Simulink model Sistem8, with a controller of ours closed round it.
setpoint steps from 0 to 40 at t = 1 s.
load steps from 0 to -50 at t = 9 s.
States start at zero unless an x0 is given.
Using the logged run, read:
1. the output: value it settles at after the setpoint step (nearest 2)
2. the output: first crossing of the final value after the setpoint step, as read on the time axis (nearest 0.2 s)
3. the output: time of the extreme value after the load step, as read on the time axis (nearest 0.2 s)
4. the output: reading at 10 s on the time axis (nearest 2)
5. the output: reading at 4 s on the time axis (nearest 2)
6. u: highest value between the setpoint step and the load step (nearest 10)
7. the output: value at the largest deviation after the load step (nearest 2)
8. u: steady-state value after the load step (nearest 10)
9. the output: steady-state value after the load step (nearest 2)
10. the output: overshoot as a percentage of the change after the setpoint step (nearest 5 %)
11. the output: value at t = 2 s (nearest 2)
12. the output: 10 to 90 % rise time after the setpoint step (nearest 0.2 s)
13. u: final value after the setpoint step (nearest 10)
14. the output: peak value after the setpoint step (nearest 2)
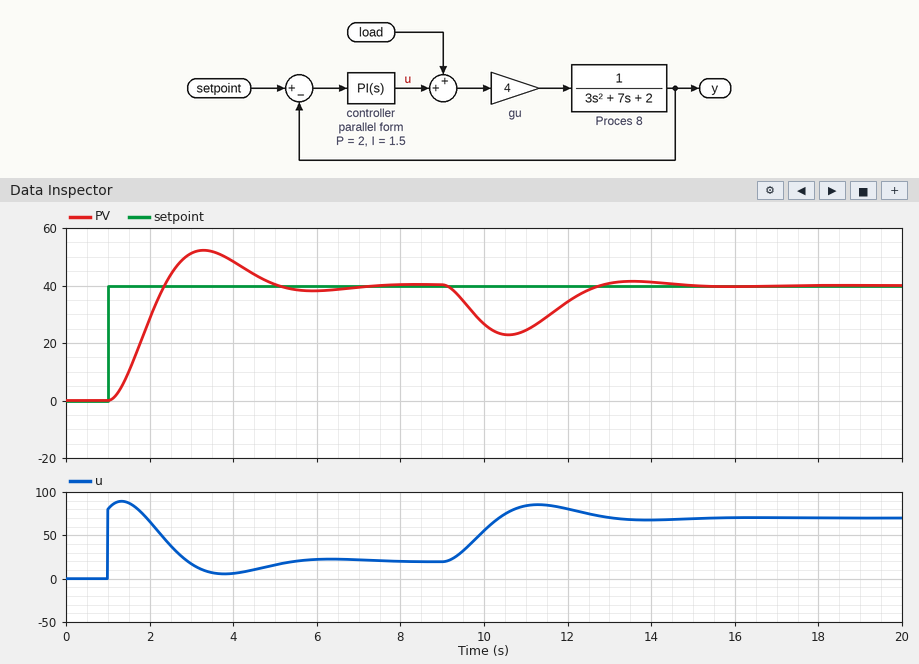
40
2.4 s
10.6 s
26
48
90
22
70
40
30 %
28
1.0 s
20
52
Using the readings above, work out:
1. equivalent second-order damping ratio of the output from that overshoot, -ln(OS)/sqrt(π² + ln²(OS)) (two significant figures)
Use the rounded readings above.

0.36
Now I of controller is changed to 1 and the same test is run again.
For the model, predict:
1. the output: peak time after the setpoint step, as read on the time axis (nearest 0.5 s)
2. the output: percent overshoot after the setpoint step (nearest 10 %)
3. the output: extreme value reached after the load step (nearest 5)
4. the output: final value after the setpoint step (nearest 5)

3.5 s
20 %
20
40
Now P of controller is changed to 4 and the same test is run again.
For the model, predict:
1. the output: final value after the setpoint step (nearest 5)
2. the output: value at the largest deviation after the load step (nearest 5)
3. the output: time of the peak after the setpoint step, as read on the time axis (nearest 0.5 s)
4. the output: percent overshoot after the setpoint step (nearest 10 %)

40
30
2.5 s
20 %
